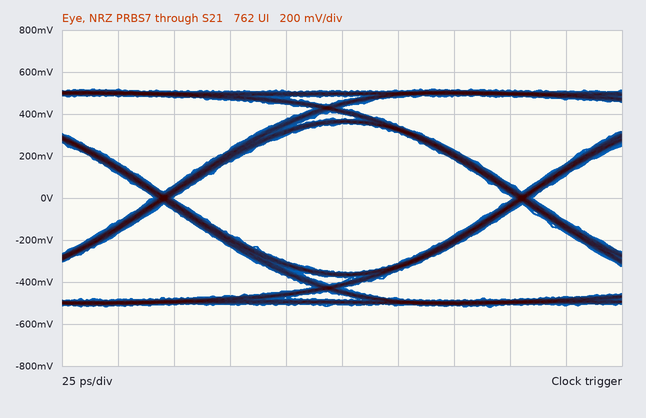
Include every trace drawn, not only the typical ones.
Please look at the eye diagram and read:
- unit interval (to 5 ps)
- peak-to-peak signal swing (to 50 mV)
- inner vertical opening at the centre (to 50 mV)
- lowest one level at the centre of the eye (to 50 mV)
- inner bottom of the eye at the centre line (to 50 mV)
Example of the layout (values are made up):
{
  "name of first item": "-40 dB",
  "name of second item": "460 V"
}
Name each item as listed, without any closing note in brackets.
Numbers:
{
  "unit interval": "160 ps",
  "peak-to-peak signal swing": "1.05 V",
  "inner vertical opening at the centre": "700 mV",
  "lowest one level at the centre of the eye": "350 mV",
  "inner bottom of the eye at the centre line": "-350 mV"
}
